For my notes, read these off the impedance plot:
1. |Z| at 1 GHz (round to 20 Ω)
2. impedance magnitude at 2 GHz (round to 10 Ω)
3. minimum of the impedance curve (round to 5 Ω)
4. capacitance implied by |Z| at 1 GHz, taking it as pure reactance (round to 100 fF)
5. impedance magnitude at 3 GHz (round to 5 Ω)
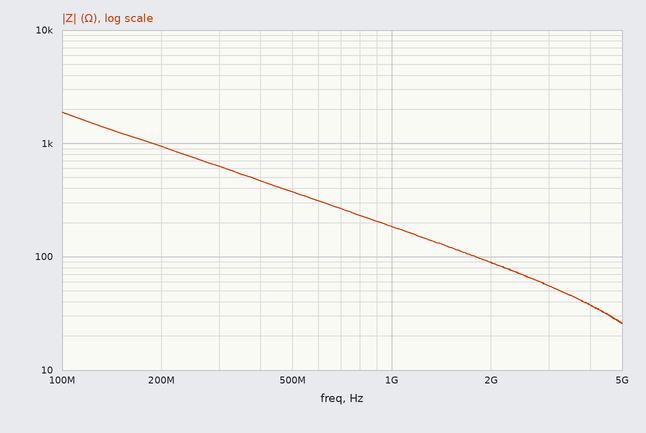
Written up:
180 Ω
90 Ω
25 Ω
900 fF
55 Ω
